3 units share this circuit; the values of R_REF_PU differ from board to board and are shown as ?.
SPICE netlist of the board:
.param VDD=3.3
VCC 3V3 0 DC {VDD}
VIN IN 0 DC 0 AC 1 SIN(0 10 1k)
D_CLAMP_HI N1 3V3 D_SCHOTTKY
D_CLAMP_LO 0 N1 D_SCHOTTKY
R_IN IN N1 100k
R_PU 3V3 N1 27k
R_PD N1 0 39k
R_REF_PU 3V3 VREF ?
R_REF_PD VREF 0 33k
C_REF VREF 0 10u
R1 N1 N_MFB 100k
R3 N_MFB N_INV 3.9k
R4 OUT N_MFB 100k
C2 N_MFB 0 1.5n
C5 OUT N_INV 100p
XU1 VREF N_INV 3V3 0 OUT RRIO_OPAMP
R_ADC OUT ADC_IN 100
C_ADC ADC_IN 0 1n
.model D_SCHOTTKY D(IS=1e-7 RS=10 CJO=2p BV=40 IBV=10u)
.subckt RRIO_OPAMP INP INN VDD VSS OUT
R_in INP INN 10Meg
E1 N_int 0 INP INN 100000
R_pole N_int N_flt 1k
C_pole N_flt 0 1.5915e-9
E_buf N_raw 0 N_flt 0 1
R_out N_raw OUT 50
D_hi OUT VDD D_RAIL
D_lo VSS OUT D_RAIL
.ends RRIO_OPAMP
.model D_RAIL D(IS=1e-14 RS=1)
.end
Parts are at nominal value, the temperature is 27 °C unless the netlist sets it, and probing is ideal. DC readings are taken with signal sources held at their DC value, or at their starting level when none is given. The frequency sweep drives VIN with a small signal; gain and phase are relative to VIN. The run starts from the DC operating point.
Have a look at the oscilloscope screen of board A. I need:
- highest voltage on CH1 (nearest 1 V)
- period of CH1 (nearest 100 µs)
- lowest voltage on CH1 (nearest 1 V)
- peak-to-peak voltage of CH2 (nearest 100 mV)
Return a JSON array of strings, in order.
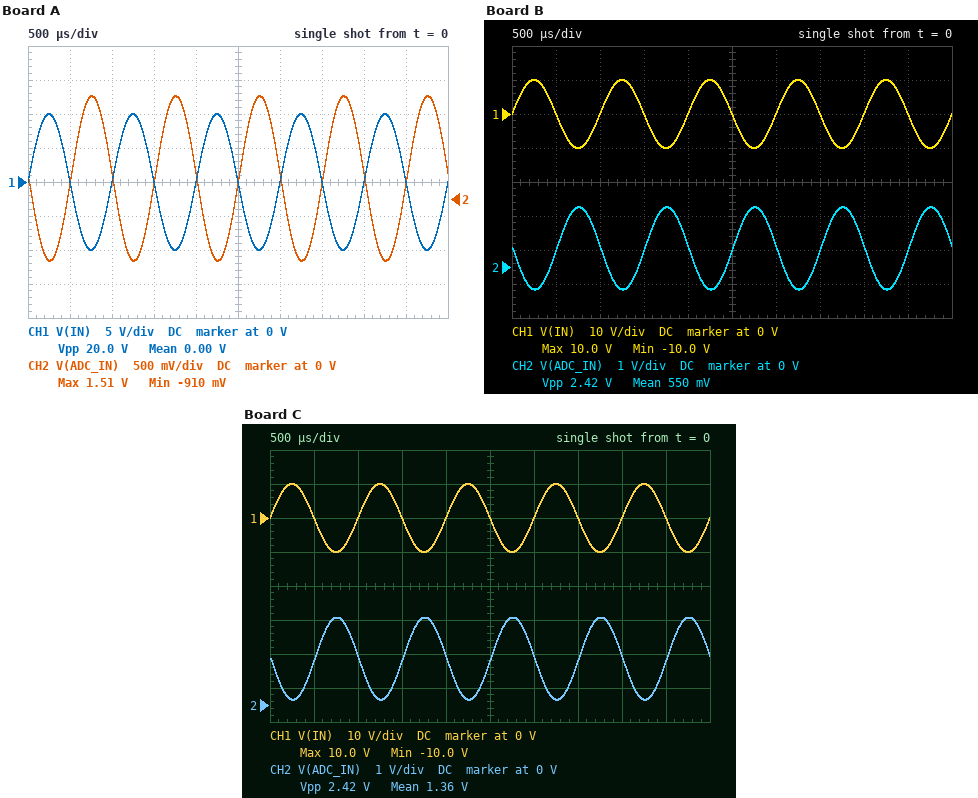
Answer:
["10 V", "1.0 ms", "-10 V", "2.4 V"]
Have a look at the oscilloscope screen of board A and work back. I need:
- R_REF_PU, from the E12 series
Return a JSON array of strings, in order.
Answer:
["82 kΩ"]
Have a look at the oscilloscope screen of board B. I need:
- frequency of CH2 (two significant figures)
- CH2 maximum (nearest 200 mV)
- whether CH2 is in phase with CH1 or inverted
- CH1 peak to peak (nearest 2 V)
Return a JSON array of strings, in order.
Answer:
["1.0 kHz", "1.8 V", "inverted", "20 V"]
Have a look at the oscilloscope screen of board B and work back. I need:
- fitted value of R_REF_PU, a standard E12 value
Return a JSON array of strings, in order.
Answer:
["68 kΩ"]
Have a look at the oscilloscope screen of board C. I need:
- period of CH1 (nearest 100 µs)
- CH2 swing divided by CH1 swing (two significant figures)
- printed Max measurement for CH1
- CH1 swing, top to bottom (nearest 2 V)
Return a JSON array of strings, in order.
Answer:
["1.0 ms", "0.12", "10.0 V", "20 V"]
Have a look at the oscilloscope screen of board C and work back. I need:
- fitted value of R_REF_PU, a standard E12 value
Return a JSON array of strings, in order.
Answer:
["39 kΩ"]
